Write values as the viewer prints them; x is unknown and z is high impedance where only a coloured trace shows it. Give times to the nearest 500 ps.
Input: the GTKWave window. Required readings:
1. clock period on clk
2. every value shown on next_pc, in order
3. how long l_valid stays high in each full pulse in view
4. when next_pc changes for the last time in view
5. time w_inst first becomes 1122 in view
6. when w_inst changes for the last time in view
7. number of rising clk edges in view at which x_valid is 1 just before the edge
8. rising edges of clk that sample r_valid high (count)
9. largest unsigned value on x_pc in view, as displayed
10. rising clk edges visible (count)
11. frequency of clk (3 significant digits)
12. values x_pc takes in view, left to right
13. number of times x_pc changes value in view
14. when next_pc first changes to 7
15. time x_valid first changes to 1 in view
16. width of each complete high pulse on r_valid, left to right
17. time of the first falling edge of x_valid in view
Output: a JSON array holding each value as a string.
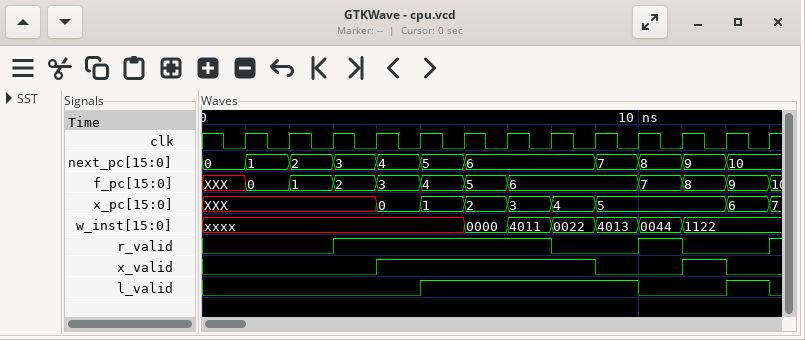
["1000 ps", "0, 1, 2, 3, 4, 5, 6, 7, 8, 9, 10", "5000 ps, 1000 ps", "12000 ps", "11000 ps", "11000 ps", "6", "6", "7", "13", "1.00 GHz", "XXX, 0, 1, 2, 3, 4, 5, 6, 7", "8", "9000 ps", "4000 ps", "5000 ps, 1000 ps", "9000 ps"]
